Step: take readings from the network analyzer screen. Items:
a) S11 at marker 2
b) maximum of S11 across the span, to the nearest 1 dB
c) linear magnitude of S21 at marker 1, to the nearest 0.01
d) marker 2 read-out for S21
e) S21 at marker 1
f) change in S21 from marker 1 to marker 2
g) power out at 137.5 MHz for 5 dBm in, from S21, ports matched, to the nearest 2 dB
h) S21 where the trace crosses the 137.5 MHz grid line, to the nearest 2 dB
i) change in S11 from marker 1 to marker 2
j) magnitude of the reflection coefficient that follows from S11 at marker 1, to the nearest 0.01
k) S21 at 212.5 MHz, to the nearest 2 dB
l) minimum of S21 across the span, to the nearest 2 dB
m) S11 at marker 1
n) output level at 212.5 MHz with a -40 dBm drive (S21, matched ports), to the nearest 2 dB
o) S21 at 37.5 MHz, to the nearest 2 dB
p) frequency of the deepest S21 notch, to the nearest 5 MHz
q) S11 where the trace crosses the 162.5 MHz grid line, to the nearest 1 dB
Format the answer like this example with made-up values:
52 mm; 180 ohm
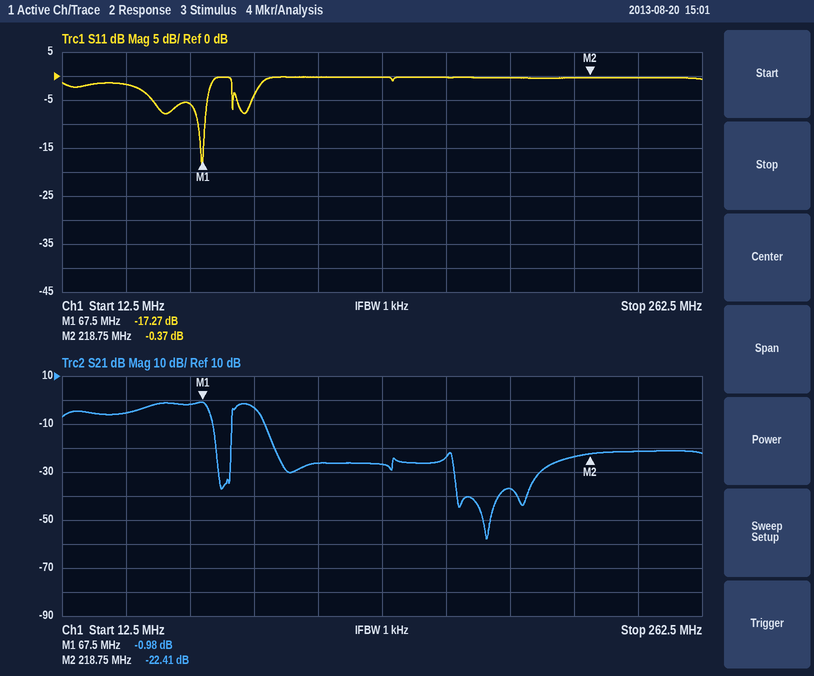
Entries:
-0.37 dB; 0 dB; 0.89; -22.41 dB; -0.98 dB; -21.43 dB; -22 dBm; -26 dB; 16.90 dB; 0.14; -24 dB; -58 dB; -17.27 dB; -64 dBm; -6 dB; 180 MHz; 0 dB
